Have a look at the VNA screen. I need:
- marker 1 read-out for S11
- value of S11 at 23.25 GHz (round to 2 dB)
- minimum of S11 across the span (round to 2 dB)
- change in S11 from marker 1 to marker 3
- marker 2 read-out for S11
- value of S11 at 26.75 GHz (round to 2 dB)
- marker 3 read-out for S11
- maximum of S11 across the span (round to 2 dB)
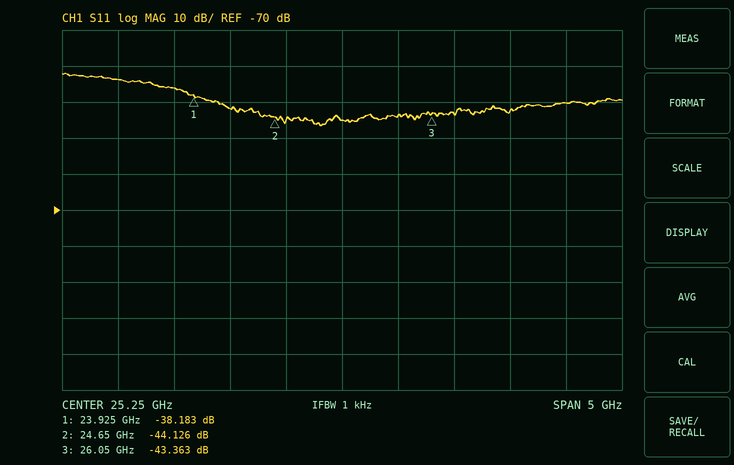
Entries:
-38.183 dB
-34 dB
-46 dB
-5.180 dB
-44.126 dB
-42 dB
-43.363 dB
-32 dB
